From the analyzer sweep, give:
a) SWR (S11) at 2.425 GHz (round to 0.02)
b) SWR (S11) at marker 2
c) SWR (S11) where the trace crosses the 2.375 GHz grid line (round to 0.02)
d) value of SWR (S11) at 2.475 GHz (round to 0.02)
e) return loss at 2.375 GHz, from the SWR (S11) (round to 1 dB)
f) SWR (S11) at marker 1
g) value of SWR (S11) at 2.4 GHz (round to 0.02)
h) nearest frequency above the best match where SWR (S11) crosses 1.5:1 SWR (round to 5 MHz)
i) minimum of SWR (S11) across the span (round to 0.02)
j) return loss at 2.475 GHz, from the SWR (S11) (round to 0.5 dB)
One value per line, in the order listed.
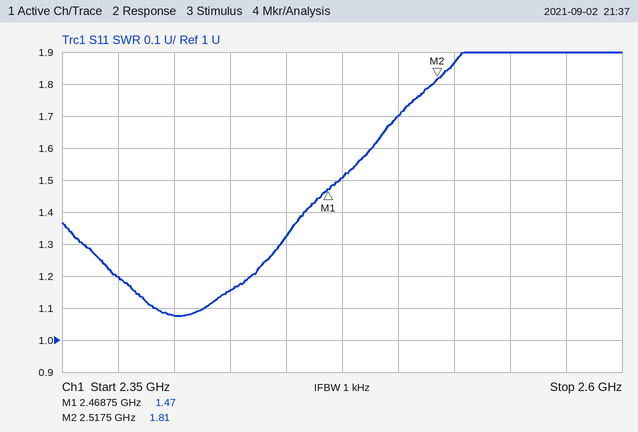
1.16
1.81
1.20
1.50
21 dB
1.47
1.08
2.475 GHz
1.08
14.0 dB
